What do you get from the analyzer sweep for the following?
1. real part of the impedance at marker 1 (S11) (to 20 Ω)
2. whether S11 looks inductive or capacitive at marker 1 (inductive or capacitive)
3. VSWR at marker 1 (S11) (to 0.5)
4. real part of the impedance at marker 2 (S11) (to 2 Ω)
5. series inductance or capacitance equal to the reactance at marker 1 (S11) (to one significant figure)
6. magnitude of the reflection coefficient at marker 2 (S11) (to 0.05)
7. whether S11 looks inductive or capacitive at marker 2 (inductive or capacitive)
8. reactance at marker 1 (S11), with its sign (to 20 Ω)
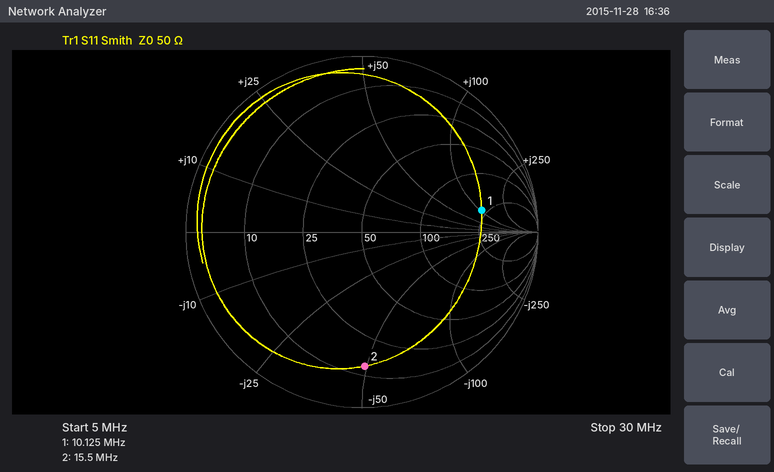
220 Ω
inductive
5.5
14 Ω
2 µH
0.75
capacitive
+100 Ω
